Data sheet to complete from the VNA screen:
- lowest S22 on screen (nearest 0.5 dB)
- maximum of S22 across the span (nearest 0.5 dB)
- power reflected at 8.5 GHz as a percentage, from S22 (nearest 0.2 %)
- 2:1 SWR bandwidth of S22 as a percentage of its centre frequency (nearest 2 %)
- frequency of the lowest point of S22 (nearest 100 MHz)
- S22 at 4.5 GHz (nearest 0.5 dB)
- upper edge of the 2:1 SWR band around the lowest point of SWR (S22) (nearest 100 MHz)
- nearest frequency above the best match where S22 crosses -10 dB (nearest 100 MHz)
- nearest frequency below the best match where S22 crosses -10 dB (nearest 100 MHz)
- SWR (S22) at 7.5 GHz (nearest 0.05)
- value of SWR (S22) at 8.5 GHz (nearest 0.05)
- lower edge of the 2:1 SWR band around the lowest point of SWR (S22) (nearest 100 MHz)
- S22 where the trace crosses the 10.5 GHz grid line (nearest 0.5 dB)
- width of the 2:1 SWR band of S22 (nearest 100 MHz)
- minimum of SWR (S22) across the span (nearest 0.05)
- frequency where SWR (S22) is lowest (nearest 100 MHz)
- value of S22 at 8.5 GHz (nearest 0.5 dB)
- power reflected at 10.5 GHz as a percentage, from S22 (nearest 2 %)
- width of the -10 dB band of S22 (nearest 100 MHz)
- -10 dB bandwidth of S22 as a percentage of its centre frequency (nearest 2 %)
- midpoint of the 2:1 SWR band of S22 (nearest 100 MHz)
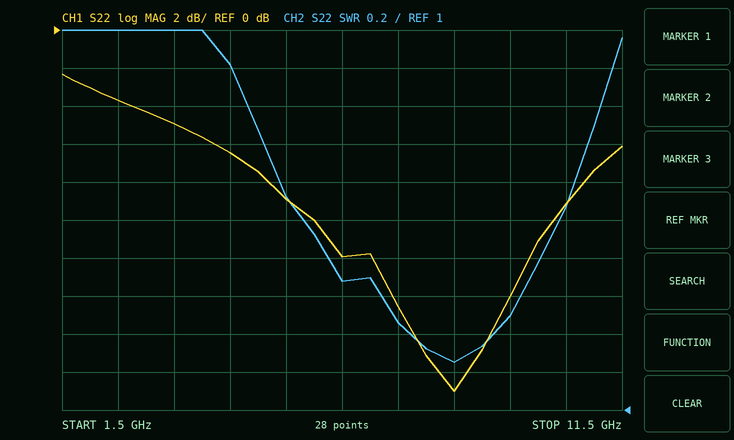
-19.0 dB
-2.5 dB
1.2 %
56 %
8.5 GHz
-6.5 dB
10.4 GHz
10.3 GHz
6.0 GHz
1.45
1.25
5.8 GHz
-9.0 dB
4.6 GHz
1.25
8.5 GHz
-19.0 dB
12 %
4.3 GHz
52 %
8.1 GHz
